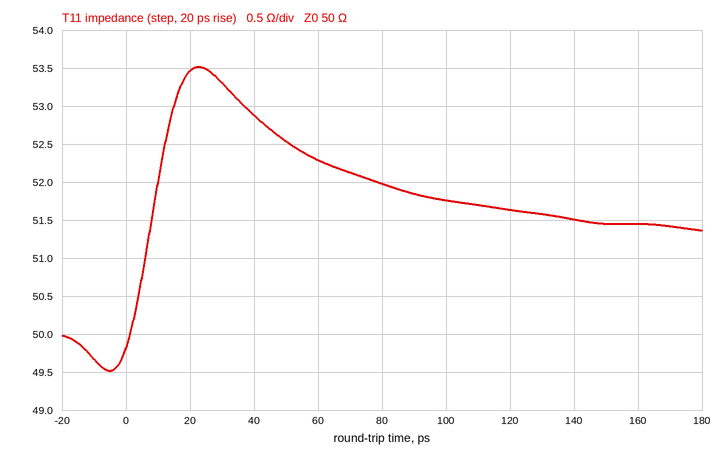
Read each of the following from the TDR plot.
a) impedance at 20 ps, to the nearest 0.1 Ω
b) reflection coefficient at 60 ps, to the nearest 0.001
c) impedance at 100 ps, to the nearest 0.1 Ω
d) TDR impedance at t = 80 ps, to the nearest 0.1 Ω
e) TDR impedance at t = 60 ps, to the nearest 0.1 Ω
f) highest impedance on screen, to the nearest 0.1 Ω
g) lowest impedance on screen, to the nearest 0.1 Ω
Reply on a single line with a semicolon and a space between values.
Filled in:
53.5 Ω; +0.022; 51.8 Ω; 52.0 Ω; 52.3 Ω; 53.5 Ω; 49.5 Ω
